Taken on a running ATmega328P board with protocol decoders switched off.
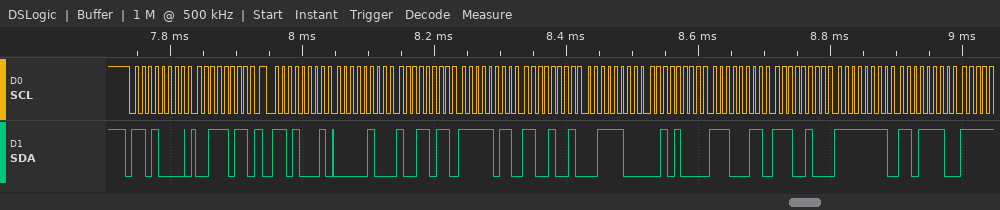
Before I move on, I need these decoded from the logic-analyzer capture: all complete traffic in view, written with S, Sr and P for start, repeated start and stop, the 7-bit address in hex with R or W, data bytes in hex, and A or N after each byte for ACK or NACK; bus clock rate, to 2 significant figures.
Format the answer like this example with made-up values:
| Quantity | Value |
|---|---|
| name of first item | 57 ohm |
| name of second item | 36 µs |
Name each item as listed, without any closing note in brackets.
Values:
| Quantity | Value |
|---|---|
| all complete traffic in view, written with S, Sr and P for start, repeated start and stop, the 7-bit address in hex with R or W, data bytes in hex, and A or N after each byte for ACK or NACK | S 68W A 3B A Sr 68R A 04 A 9B A FB A C9 A 3C A 28 A E3 A E4 A FF A DE A |
| bus clock rate, to 2 significant figures | 100 kHz |
